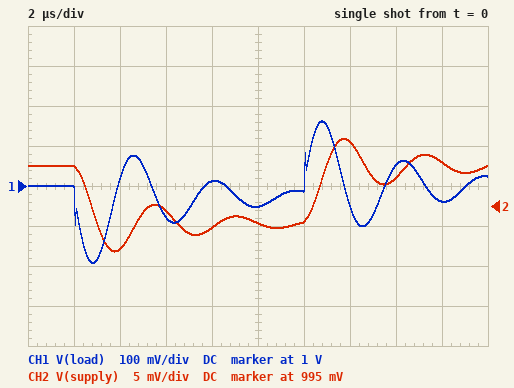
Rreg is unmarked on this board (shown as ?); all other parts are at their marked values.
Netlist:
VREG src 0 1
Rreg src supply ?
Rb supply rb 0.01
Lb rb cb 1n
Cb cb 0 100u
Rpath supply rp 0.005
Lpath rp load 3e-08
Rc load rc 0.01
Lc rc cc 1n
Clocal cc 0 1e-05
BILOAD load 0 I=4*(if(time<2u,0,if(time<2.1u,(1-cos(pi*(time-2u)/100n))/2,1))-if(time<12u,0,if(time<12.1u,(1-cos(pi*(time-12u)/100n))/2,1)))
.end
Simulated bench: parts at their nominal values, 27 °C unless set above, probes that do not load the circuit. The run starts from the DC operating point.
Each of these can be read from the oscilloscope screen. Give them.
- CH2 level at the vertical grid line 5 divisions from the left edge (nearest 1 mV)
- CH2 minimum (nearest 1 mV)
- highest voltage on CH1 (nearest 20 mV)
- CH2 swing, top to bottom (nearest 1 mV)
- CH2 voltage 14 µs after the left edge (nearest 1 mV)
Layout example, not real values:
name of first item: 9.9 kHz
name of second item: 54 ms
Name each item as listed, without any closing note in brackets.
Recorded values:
CH2 level at the vertical grid line 5 divisions from the left edge: 993 mV
CH2 minimum: 989 mV
highest voltage on CH1: 1.16 V
CH2 swing, top to bottom: 14 mV
CH2 voltage 14 µs after the left edge: 1.003 V
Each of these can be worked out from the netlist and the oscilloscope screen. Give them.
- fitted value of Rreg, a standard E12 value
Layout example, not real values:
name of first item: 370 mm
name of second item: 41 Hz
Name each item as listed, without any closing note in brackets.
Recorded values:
fitted value of Rreg, a standard E12 value: 1.8 mΩ
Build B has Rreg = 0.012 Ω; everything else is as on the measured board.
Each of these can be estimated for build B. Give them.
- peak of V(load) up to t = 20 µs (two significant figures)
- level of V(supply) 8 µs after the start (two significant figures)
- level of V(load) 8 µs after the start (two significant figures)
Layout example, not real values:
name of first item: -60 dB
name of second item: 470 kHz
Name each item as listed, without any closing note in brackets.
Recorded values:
peak of V(load) up to t = 20 µs: 1.1 V
level of V(supply) 8 µs after the start: 950 mV
level of V(load) 8 µs after the start: 960 mV
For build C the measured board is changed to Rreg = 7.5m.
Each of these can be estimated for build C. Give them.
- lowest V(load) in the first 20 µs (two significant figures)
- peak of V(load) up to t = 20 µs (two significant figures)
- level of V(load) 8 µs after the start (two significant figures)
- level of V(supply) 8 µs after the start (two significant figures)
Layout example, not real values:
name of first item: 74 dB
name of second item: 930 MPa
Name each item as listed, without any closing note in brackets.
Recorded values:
lowest V(load) in the first 20 µs: 800 mV
peak of V(load) up to t = 20 µs: 1.1 V
level of V(load) 8 µs after the start: 980 mV
level of V(supply) 8 µs after the start: 970 mV
